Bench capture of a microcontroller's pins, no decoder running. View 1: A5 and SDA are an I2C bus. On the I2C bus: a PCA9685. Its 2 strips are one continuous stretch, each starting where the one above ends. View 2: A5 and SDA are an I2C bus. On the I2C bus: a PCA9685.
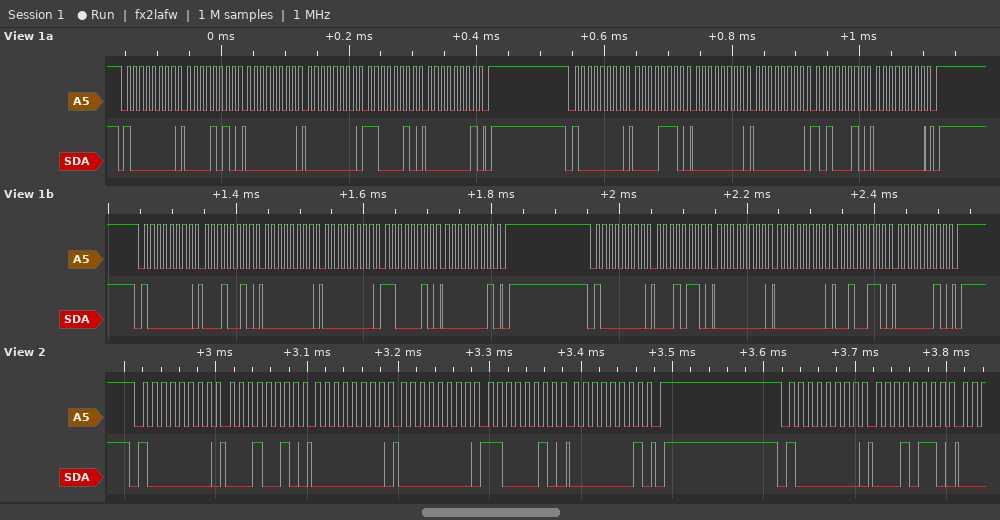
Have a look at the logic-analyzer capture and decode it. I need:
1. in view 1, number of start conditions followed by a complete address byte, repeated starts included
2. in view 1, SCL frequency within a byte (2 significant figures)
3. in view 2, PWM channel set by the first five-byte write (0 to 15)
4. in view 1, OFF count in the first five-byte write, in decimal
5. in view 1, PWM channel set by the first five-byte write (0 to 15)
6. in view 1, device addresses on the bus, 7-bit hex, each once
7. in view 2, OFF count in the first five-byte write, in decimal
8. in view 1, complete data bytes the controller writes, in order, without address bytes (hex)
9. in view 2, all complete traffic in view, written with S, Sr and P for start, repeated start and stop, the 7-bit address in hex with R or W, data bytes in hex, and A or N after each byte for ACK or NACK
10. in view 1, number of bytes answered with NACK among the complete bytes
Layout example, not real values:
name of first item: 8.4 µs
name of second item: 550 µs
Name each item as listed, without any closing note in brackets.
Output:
in view 1, number of start conditions followed by a complete address byte, repeated starts included: 4
in view 1, SCL frequency within a byte: 100 kHz
in view 2, PWM channel set by the first five-byte write: 3
in view 1, OFF count in the first five-byte write, in decimal: 450
in view 1, PWM channel set by the first five-byte write: 1
in view 1, device addresses on the bus, 7-bit hex, each once: 0x40
in view 2, OFF count in the first five-byte write, in decimal: 450
in view 1, complete data bytes the controller writes, in order, without address bytes: 0A 00 00 C2 01 0E 00 00 A2 00 12 00 00 C2 01 16 00 00 26 02
in view 2, all complete traffic in view, written with S, Sr and P for start, repeated start and stop, the 7-bit address in hex with R or W, data bytes in hex, and A or N after each byte for ACK or NACK: S 40W A 12 A 00 A 00 A C2 A 01 A P S 40W A 16 A
in view 1, number of bytes answered with NACK among the complete bytes: 0
